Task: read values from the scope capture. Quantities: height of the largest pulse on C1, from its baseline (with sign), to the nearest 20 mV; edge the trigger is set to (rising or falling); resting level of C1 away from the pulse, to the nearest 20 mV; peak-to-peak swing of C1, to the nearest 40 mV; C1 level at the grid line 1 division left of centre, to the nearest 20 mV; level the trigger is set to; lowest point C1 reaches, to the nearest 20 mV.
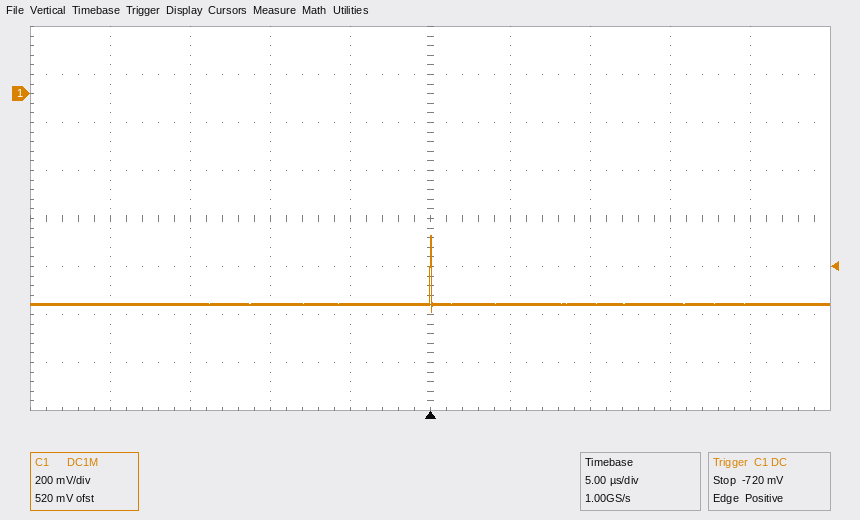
+280 mV
rising
-880 mV
320 mV
-880 mV
-720 mV
-900 mV
